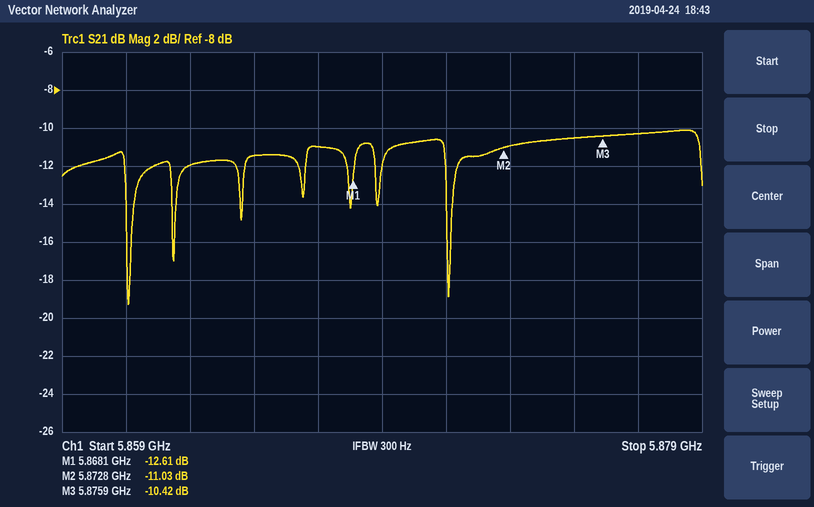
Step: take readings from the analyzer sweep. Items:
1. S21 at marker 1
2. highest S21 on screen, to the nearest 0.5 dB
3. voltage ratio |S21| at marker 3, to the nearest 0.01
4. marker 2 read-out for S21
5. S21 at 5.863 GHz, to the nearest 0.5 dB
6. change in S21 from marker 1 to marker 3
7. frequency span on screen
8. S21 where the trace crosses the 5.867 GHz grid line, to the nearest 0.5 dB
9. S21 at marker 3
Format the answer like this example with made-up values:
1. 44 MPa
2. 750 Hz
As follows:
1. -12.61 dB
2. -10.0 dB
3. 0.30
4. -11.03 dB
5. -12.0 dB
6. 2.19 dB
7. 20 MHz
8. -11.0 dB
9. -10.42 dB
